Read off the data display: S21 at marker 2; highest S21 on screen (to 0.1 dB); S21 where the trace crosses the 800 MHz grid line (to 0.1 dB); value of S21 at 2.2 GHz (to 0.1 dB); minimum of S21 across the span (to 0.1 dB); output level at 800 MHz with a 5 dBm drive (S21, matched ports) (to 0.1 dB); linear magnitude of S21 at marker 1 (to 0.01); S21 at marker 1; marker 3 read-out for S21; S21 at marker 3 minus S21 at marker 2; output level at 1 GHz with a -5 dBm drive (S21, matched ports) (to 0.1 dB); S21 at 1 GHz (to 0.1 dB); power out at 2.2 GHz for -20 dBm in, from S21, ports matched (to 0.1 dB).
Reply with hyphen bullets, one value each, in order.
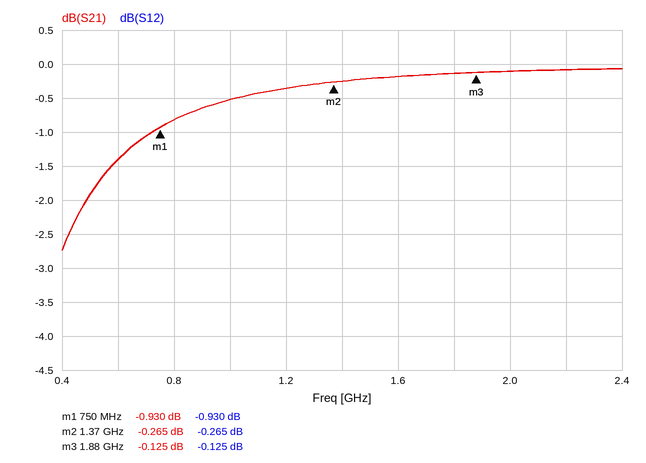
- -0.265 dB
- -0.1 dB
- -0.8 dB
- -0.1 dB
- -2.7 dB
- 4.2 dBm
- 0.90
- -0.930 dB
- -0.125 dB
- 0.140 dB
- -5.5 dBm
- -0.5 dB
- -20.1 dBm
